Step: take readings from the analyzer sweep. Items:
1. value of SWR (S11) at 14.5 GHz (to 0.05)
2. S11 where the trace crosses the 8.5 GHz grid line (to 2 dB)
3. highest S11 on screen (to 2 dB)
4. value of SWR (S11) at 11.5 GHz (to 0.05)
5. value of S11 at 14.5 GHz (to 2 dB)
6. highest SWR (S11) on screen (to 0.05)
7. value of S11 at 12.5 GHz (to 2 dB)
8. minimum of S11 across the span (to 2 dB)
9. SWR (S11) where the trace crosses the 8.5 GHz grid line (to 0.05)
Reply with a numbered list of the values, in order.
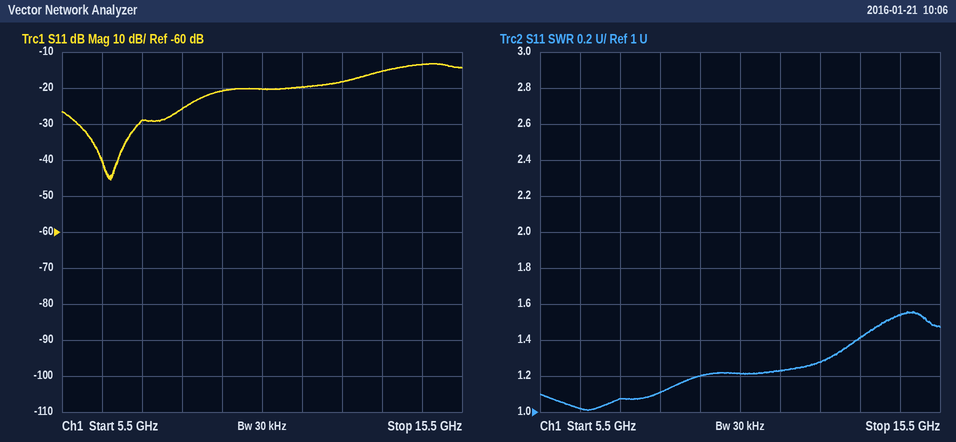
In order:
1. 1.55
2. -26 dB
3. -14 dB
4. 1.25
5. -14 dB
6. 1.55
7. -18 dB
8. -46 dB
9. 1.10
